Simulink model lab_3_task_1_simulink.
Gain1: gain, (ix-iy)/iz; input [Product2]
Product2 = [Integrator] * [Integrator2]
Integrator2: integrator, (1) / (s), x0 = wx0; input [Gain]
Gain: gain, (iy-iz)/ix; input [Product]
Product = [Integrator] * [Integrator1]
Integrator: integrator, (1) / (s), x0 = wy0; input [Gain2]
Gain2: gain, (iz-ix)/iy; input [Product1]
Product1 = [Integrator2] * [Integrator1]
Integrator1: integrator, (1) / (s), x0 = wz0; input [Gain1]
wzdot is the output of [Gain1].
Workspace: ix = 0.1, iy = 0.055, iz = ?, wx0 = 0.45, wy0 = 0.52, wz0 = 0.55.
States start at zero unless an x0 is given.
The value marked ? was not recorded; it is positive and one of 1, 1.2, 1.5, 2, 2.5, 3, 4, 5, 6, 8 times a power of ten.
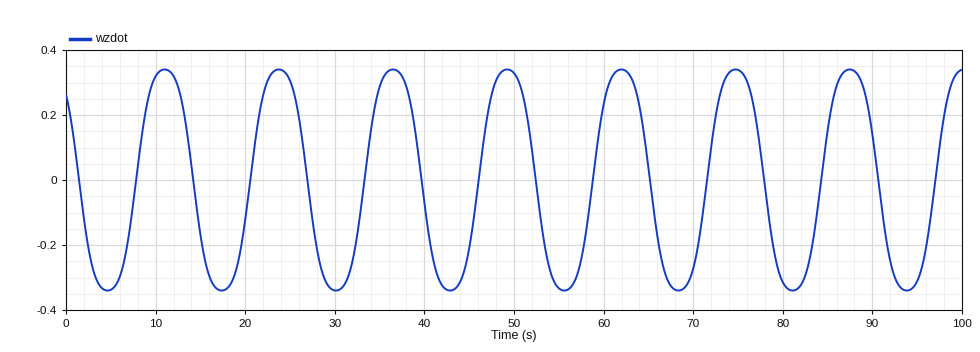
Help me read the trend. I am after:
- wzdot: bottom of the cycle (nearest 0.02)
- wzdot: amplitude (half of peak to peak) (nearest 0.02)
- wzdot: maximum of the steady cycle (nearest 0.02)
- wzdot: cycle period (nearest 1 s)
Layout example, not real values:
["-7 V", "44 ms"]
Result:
["-0.34", "0.34", "0.34", "13 s"]
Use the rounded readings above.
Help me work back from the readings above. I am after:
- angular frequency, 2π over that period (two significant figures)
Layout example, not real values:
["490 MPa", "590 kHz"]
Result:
["0.48 rad/s"]
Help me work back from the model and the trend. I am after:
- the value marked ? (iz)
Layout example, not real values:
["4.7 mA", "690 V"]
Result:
["0.04"]
